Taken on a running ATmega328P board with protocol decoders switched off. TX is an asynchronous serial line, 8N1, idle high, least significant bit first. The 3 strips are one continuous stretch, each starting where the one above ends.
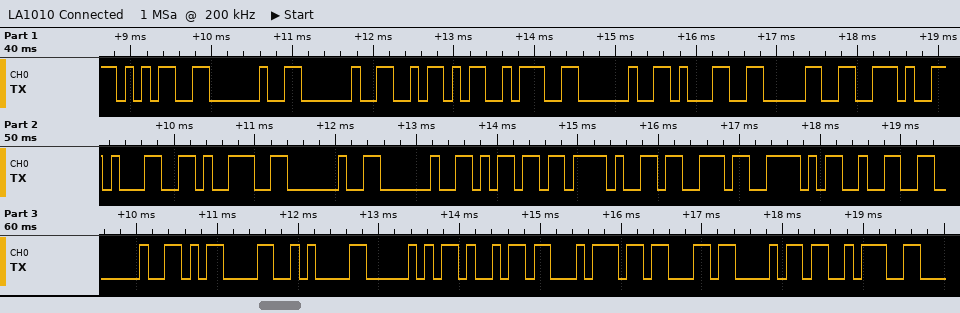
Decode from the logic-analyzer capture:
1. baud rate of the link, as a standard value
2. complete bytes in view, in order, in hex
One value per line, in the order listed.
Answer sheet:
9600 baud
35 20 20 5A 3A 20 31 30 2E 31 39 20 20 6D 2F 73 5E 32 20 0D 0A 50 69 74 63 68 3A
